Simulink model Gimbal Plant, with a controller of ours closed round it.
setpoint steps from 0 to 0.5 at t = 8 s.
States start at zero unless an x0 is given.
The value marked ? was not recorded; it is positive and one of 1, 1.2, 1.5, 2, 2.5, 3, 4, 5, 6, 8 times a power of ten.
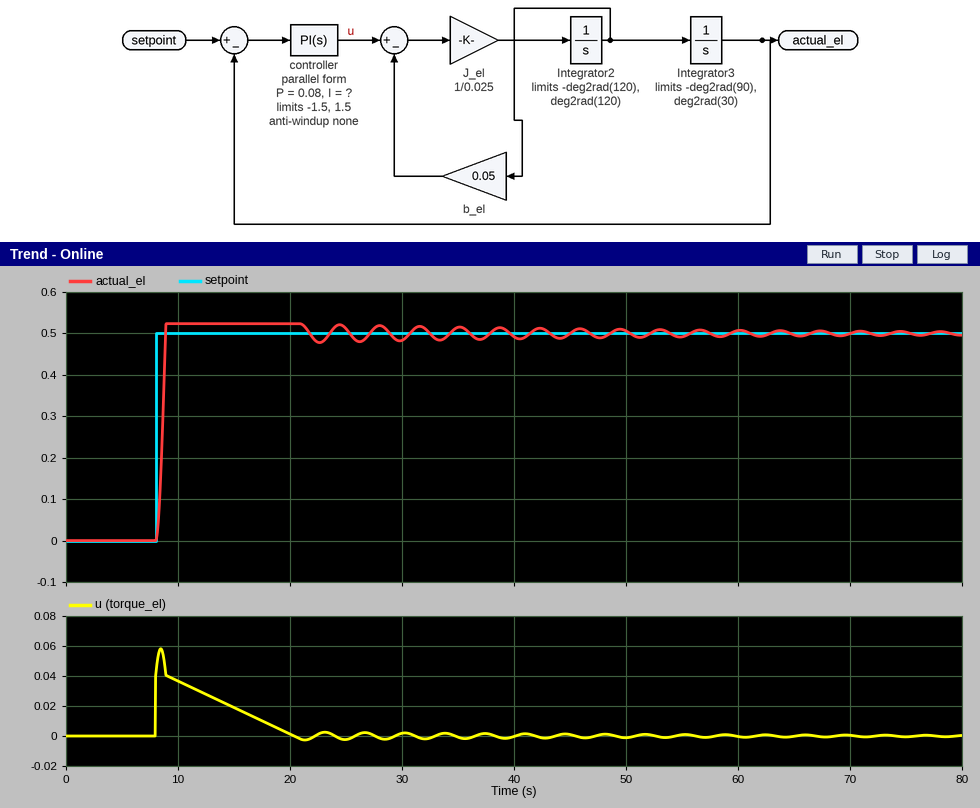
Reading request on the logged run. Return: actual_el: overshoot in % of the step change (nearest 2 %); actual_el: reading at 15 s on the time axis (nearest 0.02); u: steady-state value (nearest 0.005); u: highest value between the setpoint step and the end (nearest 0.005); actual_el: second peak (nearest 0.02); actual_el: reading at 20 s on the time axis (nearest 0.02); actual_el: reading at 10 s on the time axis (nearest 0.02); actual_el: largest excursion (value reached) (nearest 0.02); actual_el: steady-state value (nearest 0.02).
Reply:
4 %
0.52
0.000
0.060
0.52
0.52
0.52
0.52
0.50
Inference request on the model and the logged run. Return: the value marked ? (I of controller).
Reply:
0.15
